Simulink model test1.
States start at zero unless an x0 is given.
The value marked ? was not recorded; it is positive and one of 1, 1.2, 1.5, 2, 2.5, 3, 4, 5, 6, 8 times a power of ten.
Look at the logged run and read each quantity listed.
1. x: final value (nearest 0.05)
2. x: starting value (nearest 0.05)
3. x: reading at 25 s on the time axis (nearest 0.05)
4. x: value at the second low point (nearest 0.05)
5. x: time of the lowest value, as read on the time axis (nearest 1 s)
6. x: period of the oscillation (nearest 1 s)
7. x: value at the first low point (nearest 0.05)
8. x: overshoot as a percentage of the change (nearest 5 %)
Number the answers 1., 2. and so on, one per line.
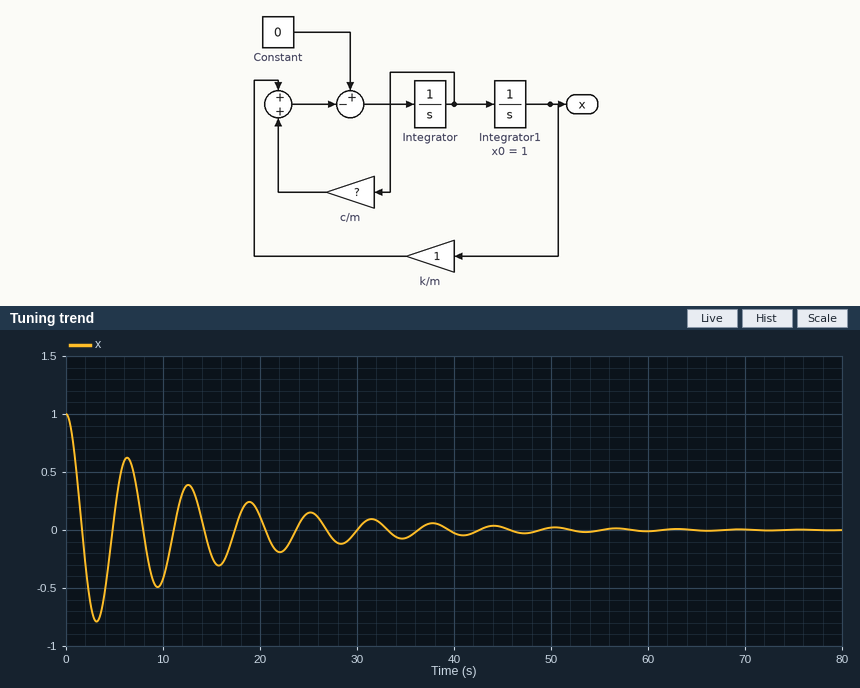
1. 0.00
2. 1.00
3. 0.15
4. -0.50
5. 3 s
6. 6 s
7. -0.80
8. 80 %
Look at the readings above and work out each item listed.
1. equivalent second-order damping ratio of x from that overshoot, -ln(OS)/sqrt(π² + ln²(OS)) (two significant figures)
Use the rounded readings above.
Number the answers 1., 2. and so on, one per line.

1. 0.071
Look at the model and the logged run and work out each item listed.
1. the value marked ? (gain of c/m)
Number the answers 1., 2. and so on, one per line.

1. 0.15
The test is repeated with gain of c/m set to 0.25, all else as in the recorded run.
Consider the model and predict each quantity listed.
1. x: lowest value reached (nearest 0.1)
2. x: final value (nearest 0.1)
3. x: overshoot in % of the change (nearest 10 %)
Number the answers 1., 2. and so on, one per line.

1. -0.7
2. 0.0
3. 70 %
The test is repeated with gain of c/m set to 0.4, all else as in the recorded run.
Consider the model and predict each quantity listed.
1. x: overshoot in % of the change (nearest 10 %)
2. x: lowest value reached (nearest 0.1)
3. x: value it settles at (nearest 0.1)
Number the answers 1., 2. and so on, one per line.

1. 50 %
2. -0.5
3. 0.0
